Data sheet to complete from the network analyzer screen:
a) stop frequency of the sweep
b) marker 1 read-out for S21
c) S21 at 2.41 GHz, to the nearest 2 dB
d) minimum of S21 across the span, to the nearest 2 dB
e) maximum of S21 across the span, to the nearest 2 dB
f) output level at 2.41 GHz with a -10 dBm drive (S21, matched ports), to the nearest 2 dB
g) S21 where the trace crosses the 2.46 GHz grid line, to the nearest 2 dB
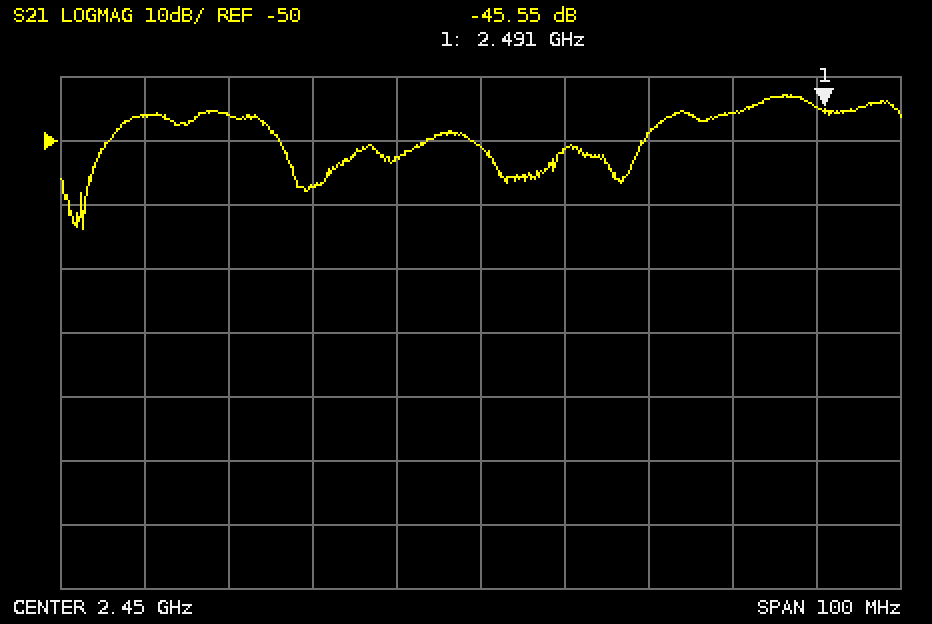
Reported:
2.5 GHz
-45.55 dB
-46 dB
-64 dB
-42 dB
-56 dBm
-52 dB
